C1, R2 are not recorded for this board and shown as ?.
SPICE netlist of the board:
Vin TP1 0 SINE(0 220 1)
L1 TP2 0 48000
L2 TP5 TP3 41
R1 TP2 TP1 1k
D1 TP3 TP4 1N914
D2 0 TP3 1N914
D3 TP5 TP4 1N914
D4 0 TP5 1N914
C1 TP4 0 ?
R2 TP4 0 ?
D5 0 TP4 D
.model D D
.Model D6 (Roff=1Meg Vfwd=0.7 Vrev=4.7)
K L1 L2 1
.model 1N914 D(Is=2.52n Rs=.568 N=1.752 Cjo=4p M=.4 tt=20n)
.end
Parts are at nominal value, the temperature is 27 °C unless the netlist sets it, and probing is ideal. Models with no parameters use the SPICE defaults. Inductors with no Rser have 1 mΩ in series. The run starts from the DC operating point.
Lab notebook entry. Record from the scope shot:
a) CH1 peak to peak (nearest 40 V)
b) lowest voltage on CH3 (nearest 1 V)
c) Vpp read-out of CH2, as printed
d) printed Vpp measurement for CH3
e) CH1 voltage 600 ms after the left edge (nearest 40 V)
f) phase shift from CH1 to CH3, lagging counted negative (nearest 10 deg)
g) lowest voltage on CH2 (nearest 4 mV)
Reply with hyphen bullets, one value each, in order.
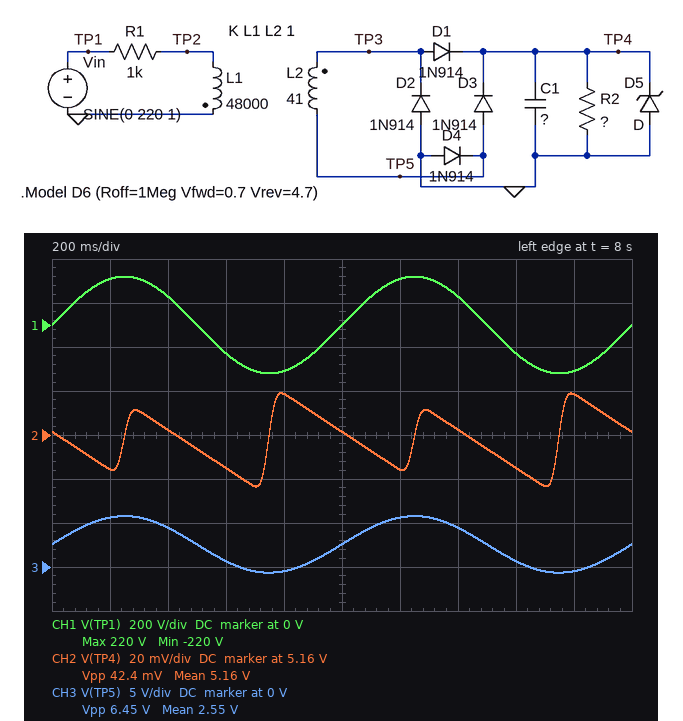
- 440 V
- -1 V
- 42.4 mV
- 6.45 V
- -120 V
- 0 deg
- 5.136 V
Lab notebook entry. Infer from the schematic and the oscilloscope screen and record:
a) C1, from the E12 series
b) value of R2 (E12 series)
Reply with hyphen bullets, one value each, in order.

- 3.3 mF
- 18 kΩ
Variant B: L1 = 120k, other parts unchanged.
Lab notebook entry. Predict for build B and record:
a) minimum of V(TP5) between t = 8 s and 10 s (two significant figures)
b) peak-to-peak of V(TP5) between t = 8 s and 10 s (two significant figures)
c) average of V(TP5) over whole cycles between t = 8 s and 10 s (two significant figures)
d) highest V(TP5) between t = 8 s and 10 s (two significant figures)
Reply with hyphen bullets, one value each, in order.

- -600 mV
- 4.1 V
- 1.4 V
- 3.5 V
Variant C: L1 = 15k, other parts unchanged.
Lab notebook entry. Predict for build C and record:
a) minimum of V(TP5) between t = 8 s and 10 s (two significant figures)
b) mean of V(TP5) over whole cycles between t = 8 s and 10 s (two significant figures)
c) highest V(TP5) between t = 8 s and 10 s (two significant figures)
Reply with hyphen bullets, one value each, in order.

- -700 mV
- 5.0 V
- 11 V
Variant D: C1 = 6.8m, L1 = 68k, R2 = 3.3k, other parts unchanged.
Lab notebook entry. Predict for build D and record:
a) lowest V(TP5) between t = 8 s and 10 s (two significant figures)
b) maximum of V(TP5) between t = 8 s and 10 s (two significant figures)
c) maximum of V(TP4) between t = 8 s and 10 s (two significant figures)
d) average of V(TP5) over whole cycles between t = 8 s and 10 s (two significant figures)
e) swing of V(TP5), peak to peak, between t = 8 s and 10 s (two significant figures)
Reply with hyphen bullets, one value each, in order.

- -700 mV
- 4.7 V
- 4.0 V
- 2.0 V
- 5.4 V
